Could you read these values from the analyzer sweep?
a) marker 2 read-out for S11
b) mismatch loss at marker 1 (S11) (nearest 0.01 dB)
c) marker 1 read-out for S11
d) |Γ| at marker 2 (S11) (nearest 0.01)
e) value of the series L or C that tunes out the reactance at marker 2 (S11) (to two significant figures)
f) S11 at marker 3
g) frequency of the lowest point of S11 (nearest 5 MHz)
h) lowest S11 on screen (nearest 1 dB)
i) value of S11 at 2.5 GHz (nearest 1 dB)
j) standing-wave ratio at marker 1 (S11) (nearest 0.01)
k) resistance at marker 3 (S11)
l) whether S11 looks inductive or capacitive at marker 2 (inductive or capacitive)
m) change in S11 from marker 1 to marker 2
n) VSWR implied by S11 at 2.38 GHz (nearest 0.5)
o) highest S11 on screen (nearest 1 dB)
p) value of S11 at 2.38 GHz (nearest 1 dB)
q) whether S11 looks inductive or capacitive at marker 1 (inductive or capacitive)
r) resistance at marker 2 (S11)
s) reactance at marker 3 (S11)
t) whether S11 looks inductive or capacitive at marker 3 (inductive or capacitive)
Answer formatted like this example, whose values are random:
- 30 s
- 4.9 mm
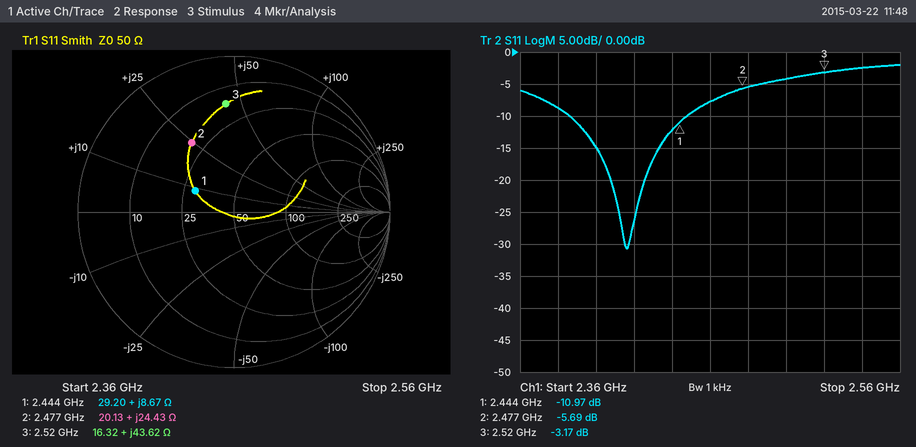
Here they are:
- -5.69 dB
- 0.36 dB
- -10.97 dB
- 0.52
- 2.6 pF
- -3.17 dB
- 2.415 GHz
- -31 dB
- -4 dB
- 1.79
- 16.32 Ω
- inductive
- 5.28 dB
- 2.0
- -2 dB
- -9 dB
- inductive
- 20.13 Ω
- +43.62 Ω
- inductive
